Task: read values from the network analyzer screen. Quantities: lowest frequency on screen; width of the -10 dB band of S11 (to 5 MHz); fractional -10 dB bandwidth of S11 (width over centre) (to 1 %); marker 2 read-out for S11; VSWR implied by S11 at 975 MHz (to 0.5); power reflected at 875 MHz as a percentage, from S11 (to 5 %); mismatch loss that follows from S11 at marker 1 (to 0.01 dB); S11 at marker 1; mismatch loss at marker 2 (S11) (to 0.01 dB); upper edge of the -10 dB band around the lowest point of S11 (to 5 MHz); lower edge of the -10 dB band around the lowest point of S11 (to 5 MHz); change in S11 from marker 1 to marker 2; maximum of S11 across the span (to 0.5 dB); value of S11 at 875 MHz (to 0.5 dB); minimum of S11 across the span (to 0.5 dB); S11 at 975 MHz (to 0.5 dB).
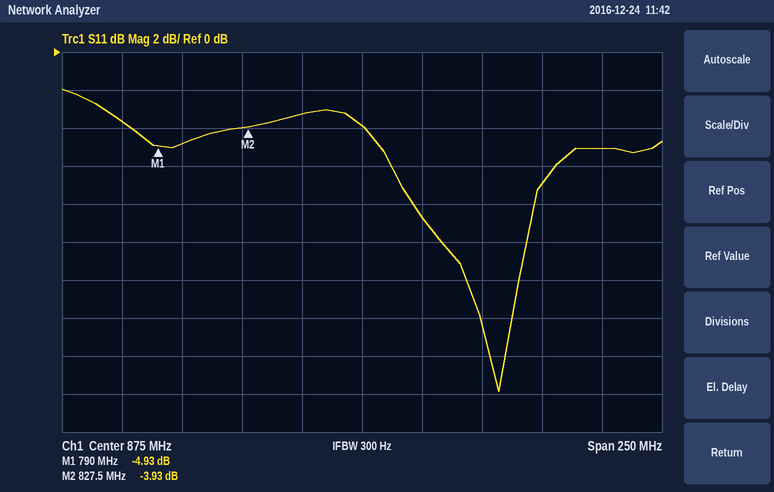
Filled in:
750 MHz
35 MHz
4 %
-3.93 dB
3.5
40 %
1.68 dB
-4.93 dB
2.25 dB
945 MHz
910 MHz
1.00 dB
-2.0 dB
-4.0 dB
-18.0 dB
-5.0 dB
